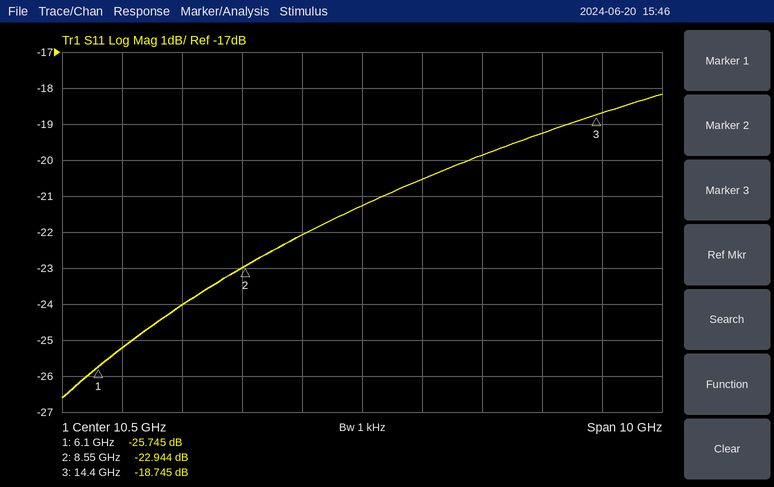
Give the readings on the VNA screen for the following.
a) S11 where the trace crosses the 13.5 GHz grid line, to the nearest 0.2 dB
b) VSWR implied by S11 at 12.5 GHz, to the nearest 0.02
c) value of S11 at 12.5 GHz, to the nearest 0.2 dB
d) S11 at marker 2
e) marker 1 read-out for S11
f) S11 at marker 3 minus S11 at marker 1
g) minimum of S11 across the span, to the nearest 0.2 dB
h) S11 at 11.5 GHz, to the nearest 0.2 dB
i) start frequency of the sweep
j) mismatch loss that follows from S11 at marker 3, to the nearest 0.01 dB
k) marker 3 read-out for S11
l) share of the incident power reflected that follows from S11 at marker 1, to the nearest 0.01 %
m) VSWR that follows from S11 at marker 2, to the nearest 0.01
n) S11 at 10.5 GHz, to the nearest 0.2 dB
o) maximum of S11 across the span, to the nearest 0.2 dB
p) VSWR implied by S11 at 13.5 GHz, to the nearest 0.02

-19.2 dB
1.22
-19.8 dB
-22.944 dB
-25.745 dB
7.000 dB
-26.6 dB
-20.6 dB
5.5 GHz
0.06 dB
-18.745 dB
0.27 %
1.15
-21.2 dB
-18.2 dB
1.24
